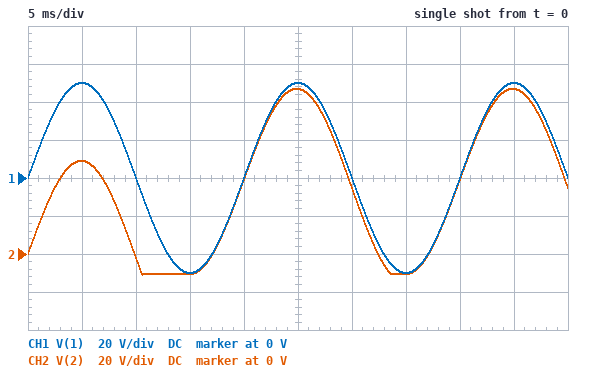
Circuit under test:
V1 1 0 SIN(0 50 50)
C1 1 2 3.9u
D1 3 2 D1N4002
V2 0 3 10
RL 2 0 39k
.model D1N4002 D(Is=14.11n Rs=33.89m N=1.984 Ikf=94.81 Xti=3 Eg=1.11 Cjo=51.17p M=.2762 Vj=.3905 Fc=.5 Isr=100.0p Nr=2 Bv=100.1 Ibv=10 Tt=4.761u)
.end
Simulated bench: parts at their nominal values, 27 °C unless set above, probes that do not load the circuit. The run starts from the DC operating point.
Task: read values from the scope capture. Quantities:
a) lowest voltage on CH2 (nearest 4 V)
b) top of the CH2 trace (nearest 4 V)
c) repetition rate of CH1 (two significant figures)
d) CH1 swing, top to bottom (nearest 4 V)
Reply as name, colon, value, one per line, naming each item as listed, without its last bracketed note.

lowest voltage on CH2: -12 V
top of the CH2 trace: 88 V
repetition rate of CH1: 50 Hz
CH1 swing, top to bottom: 100 V
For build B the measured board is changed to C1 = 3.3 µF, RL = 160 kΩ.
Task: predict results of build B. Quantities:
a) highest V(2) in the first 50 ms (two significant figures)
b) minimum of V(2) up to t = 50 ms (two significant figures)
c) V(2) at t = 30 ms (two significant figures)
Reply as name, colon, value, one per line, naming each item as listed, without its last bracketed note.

highest V(2) in the first 50 ms: 89 V
minimum of V(2) up to t = 50 ms: -11 V
V(2) at t = 30 ms: 38 V
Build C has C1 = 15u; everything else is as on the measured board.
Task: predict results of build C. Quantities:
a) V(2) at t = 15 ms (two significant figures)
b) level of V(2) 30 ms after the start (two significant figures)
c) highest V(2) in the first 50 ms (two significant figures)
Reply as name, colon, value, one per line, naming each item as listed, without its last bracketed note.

V(2) at t = 15 ms: -11 V
level of V(2) 30 ms after the start: 38 V
highest V(2) in the first 50 ms: 89 V
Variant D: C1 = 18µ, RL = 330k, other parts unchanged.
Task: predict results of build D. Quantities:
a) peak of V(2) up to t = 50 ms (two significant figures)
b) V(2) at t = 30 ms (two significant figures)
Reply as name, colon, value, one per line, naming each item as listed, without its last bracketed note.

peak of V(2) up to t = 50 ms: 89 V
V(2) at t = 30 ms: 39 V
